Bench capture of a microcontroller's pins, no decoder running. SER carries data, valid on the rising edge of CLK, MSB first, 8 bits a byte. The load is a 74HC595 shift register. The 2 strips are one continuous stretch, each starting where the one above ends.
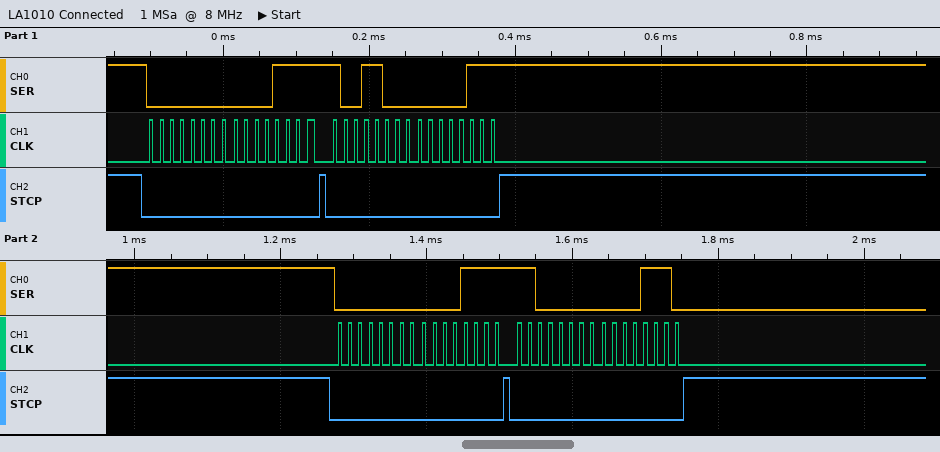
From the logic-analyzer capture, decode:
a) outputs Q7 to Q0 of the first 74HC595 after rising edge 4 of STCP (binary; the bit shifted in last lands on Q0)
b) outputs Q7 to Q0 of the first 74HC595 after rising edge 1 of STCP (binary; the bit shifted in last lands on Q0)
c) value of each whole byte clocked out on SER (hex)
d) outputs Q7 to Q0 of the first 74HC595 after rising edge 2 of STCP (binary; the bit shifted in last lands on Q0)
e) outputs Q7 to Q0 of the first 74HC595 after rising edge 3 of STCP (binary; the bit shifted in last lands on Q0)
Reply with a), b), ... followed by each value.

a) 00001110
b) 00001111
c) 00 0F 98 07 00 0F C0 0E
d) 00000111
e) 00001111
